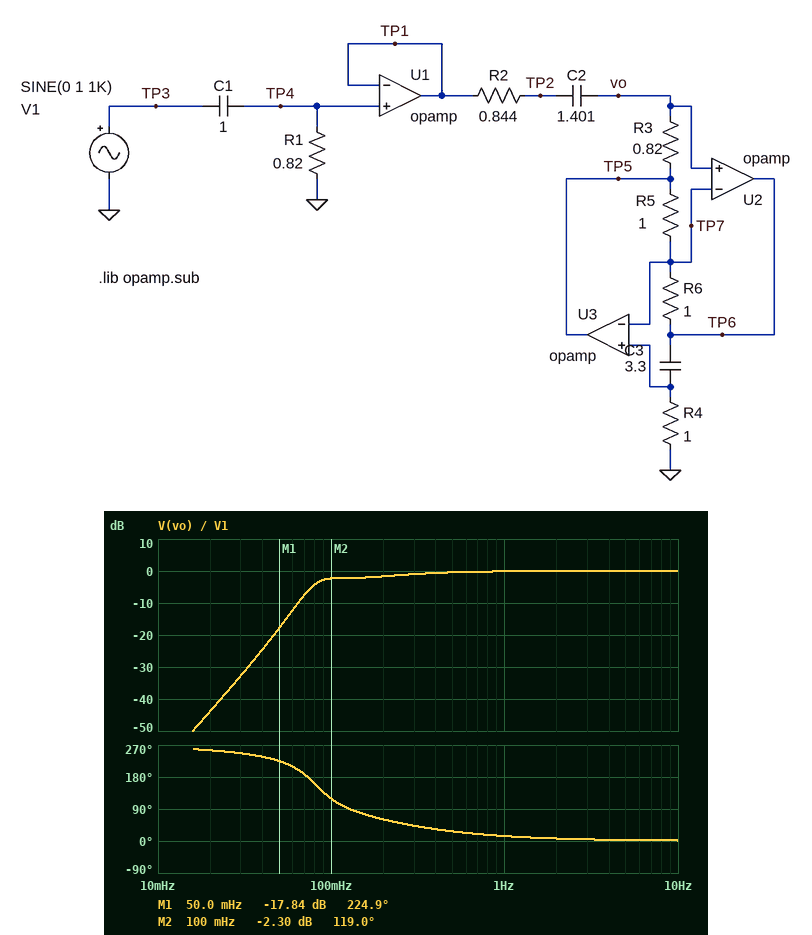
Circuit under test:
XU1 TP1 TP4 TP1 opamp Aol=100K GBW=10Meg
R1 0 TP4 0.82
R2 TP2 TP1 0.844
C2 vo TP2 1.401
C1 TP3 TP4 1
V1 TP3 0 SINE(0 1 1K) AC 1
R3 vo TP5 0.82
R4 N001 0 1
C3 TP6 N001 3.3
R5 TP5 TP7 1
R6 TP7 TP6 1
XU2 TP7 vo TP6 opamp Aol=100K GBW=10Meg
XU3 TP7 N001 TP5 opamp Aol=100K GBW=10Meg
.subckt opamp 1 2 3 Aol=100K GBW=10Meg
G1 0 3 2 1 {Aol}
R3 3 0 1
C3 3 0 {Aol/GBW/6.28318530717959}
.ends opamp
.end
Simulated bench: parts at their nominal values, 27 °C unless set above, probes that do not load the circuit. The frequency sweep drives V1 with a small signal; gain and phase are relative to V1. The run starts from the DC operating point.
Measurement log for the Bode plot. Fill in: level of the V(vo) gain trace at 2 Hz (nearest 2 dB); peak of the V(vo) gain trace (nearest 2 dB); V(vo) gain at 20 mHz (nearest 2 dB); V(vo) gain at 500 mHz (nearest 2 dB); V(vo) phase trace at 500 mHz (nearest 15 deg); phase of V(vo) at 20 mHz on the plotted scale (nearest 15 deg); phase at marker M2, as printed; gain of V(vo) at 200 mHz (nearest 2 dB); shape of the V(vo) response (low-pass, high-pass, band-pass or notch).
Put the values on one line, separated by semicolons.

0 dB; 0 dB; -44 dB; 0 dB; 30 deg; 255 deg; 119.0 deg; -2 dB; high-pass
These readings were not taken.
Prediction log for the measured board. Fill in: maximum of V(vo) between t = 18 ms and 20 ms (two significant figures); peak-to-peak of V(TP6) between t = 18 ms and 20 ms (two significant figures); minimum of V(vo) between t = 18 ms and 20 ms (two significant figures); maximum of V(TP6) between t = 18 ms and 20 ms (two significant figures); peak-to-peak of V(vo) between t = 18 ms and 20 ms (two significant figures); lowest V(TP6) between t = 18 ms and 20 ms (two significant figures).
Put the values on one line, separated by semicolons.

1.0 V; 2.0 V; -1.0 V; 1.0 V; 2.0 V; -1.0 V
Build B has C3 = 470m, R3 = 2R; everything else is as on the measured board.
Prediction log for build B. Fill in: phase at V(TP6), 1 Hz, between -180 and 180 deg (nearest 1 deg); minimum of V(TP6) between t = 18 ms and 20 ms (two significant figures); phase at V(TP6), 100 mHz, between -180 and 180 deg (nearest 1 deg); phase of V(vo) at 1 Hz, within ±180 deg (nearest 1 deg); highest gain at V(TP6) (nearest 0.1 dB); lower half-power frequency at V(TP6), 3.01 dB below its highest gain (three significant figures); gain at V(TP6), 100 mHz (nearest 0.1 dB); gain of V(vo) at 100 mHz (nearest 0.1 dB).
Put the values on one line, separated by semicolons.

1 deg; -1.0 V; 112 deg; 19 deg; 4.2 dB; 112 mHz; -0.4 dB; -11.4 dB
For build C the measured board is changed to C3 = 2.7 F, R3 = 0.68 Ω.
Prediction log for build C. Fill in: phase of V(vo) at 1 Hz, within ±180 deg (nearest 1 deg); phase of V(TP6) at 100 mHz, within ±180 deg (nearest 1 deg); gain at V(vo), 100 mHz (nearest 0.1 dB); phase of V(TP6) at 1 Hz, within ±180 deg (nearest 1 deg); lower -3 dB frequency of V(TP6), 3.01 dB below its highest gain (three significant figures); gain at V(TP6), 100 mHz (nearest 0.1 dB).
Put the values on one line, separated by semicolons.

15 deg; 121 deg; -4.1 dB; 12 deg; 98.3 mHz; -2.8 dB
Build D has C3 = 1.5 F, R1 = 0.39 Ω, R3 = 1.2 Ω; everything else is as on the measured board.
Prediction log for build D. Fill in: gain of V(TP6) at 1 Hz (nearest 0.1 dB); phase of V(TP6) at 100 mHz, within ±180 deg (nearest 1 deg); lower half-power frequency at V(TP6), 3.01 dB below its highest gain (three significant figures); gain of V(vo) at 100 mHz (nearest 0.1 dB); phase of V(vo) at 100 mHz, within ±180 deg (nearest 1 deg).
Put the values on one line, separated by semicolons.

-0.6 dB; 120 deg; 331 mHz; -9.9 dB; 167 deg
